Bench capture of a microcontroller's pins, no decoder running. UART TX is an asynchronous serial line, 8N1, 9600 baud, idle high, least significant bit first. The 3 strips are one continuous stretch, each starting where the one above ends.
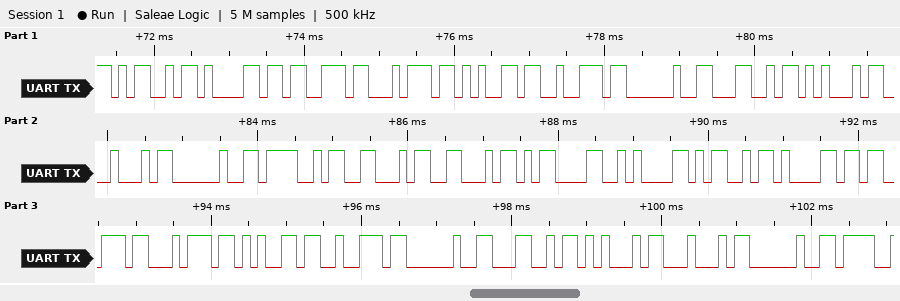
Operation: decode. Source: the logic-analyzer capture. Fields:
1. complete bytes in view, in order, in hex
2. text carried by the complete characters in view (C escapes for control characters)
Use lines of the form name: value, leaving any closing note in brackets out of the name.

complete bytes in view, in order, in hex: 4D 61 73 74 65 72 20 4C 45 44 20 4F 46 46 0D 0A 4D 61 73 74 65 72 20 4C 45 44 20
text carried by the complete characters in view: "Master LED OFF\r\nMaster LED "
